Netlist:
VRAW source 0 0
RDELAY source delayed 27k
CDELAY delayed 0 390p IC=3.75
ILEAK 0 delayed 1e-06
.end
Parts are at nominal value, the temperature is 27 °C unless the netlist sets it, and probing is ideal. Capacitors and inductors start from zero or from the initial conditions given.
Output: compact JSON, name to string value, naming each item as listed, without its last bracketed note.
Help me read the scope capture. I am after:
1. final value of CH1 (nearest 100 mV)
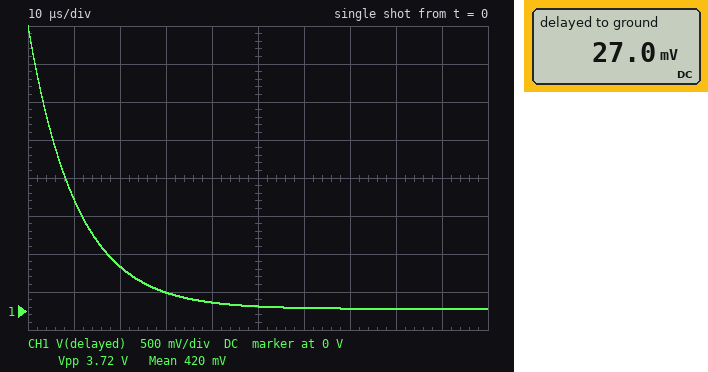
{"final value of CH1": "0 V"}
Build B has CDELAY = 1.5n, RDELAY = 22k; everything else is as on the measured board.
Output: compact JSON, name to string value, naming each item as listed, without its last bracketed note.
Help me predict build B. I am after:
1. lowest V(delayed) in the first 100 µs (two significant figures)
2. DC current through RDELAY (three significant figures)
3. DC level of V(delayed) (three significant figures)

{"lowest V(delayed) in the first 100 µs": "200 mV", "DC current through RDELAY": "1.00 µA", "DC level of V(delayed)": "22.0 mV"}
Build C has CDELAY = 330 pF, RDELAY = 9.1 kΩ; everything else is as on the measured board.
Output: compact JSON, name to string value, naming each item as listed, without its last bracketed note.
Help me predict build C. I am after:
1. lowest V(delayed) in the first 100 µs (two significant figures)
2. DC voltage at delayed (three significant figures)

{"lowest V(delayed) in the first 100 µs": "9.1 mV", "DC voltage at delayed": "9.10 mV"}
